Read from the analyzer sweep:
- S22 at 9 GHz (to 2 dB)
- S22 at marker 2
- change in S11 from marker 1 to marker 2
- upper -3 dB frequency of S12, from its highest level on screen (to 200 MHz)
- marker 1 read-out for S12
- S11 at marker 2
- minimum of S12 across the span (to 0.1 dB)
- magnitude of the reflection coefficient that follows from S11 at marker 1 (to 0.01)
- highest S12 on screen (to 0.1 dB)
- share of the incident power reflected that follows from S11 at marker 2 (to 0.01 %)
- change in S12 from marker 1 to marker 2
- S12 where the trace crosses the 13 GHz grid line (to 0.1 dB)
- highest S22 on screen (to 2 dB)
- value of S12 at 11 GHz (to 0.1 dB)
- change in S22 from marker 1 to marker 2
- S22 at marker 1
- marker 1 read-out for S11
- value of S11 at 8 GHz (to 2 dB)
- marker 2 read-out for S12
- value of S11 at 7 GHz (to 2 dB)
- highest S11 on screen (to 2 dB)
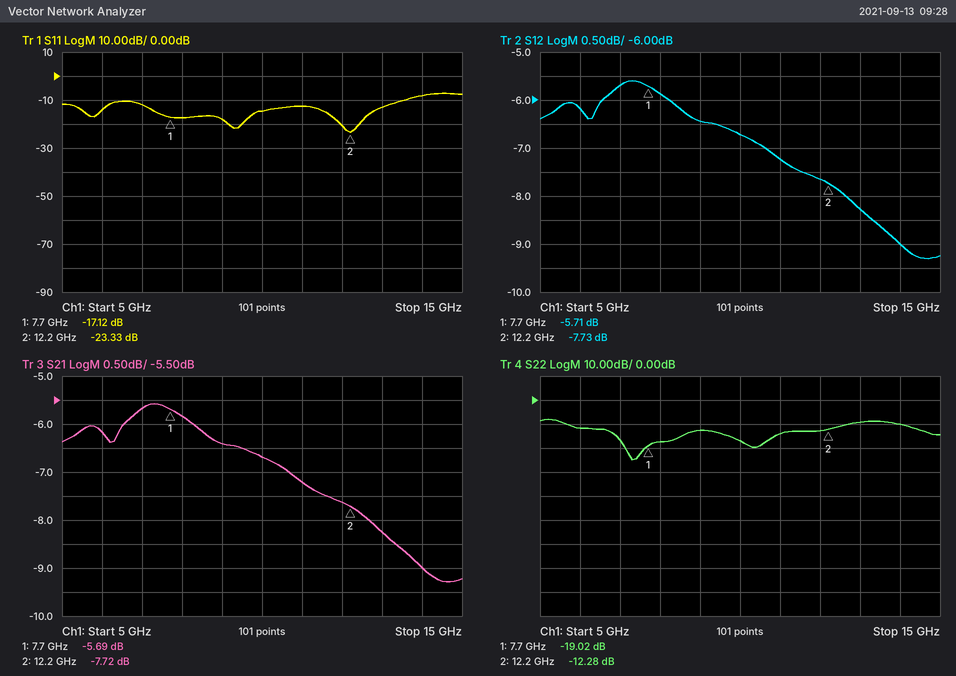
-12 dB
-12.28 dB
-6.21 dB
13.4 GHz
-5.71 dB
-23.33 dB
-9.3 dB
0.14
-5.6 dB
0.46 %
-2.02 dB
-8.3 dB
-8 dB
-7.2 dB
6.74 dB
-19.02 dB
-17.12 dB
-18 dB
-7.73 dB
-12 dB
-8 dB
